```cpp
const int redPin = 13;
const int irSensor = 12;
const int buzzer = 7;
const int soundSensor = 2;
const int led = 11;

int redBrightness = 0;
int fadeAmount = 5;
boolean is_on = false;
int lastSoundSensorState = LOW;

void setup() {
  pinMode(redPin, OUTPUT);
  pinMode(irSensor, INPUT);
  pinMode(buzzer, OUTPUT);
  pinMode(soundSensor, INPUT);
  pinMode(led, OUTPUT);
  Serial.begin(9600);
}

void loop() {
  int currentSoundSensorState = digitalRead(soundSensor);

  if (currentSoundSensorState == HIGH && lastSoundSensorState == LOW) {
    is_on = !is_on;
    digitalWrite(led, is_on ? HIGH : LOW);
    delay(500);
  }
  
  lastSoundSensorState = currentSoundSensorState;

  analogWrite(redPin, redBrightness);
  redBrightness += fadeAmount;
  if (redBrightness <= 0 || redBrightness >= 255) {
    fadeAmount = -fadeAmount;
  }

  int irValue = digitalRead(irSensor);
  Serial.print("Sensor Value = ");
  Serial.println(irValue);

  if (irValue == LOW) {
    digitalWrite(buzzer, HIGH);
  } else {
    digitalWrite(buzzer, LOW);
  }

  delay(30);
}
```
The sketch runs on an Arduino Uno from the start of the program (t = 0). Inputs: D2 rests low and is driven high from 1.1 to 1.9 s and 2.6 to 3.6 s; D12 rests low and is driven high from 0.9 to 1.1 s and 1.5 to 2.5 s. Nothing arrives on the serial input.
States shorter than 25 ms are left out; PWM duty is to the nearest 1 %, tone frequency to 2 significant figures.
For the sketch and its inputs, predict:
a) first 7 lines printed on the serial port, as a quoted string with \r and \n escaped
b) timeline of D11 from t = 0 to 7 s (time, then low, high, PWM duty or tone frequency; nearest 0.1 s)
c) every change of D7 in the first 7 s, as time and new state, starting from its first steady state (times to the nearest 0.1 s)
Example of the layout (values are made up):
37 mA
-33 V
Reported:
"Sensor Value = 0\r\nSensor Value = 0\r\nSensor Value = 0\r\nSensor Value = 0\r\nSensor Value = 0\r\nSensor Value = 0\r\nSensor Value = 0\r\n"
0 s low; 1.1 s high; 2.6 s low
0 s high; 0.9 s low; 2.5 s high
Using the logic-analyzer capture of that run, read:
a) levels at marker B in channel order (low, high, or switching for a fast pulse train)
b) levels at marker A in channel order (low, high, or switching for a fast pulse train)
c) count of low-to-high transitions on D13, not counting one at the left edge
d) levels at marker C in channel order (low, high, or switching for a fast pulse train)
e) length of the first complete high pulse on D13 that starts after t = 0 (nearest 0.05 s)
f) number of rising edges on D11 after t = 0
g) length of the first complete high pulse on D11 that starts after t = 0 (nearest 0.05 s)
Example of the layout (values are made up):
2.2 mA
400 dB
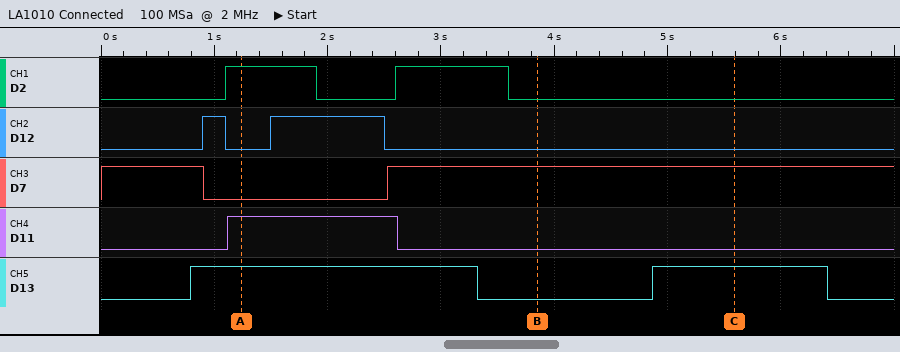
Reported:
D2 low, D12 low, D7 high, D11 low, D13 low
D2 high, D12 low, D7 low, D11 high, D13 high
2
D2 low, D12 low, D7 high, D11 low, D13 high
2.55 s
1
1.50 s
